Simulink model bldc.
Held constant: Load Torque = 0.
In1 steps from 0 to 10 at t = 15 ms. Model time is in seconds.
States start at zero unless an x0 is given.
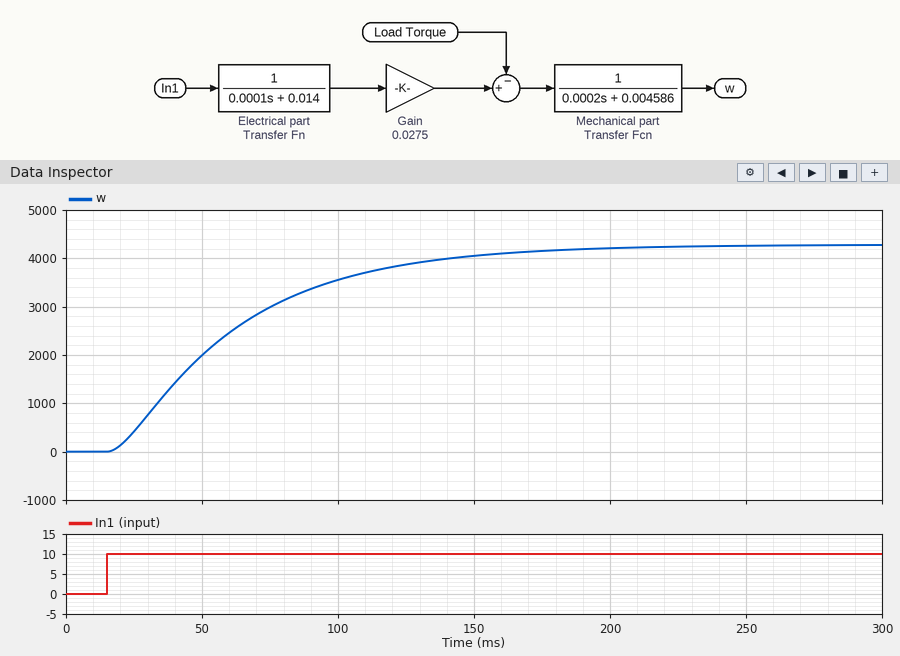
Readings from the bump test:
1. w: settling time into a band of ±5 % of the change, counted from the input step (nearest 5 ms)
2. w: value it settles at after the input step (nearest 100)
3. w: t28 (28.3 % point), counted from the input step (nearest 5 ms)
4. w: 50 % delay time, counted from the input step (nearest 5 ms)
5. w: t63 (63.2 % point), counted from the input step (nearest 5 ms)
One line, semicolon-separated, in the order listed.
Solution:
140 ms; 4300; 20 ms; 40 ms; 50 ms
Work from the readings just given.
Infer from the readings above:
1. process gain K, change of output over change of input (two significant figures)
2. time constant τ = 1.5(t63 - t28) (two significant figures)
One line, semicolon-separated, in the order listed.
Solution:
430; 45 ms
